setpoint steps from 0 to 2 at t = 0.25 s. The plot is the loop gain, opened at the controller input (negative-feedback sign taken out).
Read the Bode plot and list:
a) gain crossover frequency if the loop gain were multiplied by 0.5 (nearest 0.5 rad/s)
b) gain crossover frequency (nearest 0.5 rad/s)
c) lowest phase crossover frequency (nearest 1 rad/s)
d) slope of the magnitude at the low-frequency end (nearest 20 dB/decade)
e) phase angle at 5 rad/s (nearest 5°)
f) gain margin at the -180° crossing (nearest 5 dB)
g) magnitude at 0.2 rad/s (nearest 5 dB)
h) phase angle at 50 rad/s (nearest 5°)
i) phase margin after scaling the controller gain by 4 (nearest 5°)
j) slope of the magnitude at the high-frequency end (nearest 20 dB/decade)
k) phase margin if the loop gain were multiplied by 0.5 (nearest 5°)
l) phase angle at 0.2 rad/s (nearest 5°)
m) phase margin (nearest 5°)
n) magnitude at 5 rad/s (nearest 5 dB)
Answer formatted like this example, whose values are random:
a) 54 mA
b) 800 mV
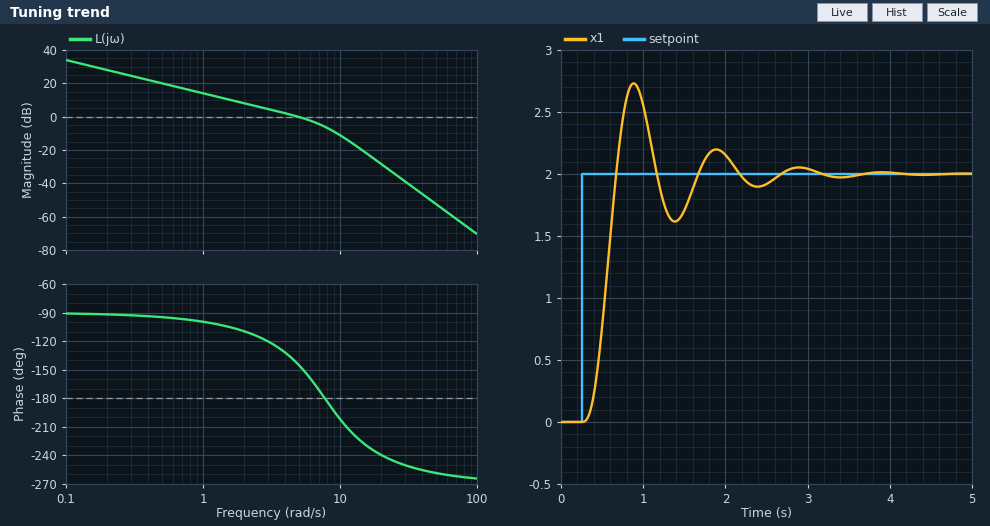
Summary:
a) 2.5 rad/s
b) 5.0 rad/s
c) 8 rad/s
d) -20 dB/decade
e) -145°
f) 5 dB
g) 30 dB
h) -260°
i) -25°
j) -60 dB/decade
k) 65°
l) -90°
m) 35°
n) 0 dB
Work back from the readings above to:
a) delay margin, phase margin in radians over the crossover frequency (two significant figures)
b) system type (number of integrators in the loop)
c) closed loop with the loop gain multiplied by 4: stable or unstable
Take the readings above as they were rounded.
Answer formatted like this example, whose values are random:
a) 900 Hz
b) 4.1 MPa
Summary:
a) 0.12 s
b) 1
c) unstable
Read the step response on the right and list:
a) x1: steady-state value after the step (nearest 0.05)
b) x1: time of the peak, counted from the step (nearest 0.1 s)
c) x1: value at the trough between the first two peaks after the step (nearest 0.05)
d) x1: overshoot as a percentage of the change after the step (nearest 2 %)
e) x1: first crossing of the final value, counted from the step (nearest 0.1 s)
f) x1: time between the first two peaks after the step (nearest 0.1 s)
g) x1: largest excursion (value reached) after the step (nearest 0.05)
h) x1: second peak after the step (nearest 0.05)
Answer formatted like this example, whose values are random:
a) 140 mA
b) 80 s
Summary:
a) 2.00
b) 0.6 s
c) 1.60
d) 36 %
e) 0.4 s
f) 1.0 s
g) 2.75
h) 2.20
